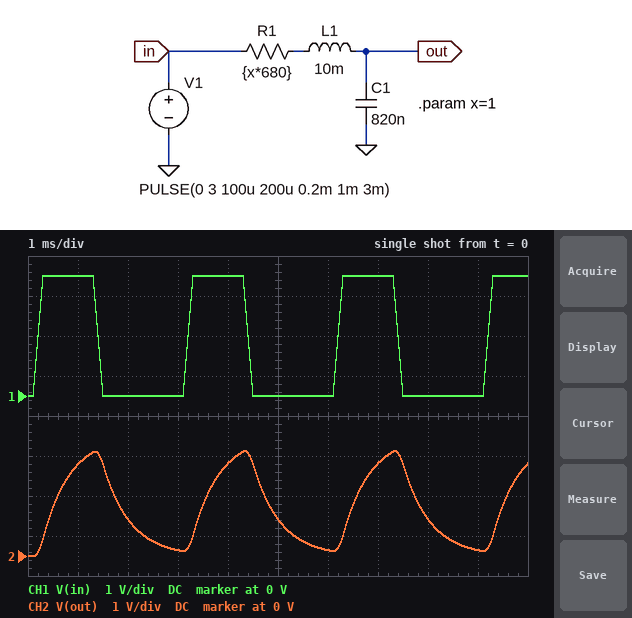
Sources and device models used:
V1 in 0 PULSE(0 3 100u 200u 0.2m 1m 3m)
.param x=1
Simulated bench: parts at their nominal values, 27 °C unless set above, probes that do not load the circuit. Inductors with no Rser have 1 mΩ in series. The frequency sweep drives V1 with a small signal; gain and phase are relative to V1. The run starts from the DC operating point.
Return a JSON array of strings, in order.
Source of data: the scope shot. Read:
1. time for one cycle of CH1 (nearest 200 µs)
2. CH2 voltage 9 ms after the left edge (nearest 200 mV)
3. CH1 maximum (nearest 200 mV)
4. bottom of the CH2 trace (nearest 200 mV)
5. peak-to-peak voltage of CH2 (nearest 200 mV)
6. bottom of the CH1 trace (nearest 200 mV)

["3.0 ms", "200 mV", "3.0 V", "0 V", "2.6 V", "0 V"]
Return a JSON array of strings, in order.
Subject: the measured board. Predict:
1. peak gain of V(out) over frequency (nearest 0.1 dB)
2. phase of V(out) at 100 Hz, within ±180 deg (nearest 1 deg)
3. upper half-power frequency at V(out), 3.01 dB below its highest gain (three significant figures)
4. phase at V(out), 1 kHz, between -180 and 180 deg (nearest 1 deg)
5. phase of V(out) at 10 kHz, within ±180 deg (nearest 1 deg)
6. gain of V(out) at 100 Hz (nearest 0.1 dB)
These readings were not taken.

["0 dB", "-19 deg", "293 Hz", "-79 deg", "-132 deg", "-0.5 dB"]
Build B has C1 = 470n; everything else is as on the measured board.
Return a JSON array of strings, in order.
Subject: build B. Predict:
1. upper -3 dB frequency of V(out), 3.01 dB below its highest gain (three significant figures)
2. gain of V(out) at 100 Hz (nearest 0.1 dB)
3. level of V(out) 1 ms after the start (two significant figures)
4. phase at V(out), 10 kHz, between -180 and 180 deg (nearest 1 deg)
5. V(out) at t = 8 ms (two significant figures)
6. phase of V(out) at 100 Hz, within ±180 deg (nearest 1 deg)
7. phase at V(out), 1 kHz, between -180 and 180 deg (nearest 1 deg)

["522 Hz", "-0.2 dB", "2.8 V", "-131 deg", "440 mV", "-11 deg", "-68 deg"]
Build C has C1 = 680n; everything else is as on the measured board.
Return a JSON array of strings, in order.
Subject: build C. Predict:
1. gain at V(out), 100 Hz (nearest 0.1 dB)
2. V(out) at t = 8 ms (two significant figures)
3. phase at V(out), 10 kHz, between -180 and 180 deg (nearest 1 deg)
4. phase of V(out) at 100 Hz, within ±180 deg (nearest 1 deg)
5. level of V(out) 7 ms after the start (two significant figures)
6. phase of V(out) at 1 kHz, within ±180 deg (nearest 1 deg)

["-0.3 dB", "760 mV", "-132 deg", "-16 deg", "2.5 V", "-76 deg"]
